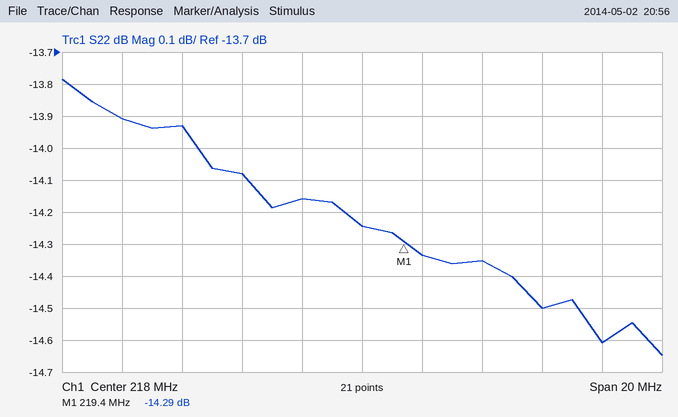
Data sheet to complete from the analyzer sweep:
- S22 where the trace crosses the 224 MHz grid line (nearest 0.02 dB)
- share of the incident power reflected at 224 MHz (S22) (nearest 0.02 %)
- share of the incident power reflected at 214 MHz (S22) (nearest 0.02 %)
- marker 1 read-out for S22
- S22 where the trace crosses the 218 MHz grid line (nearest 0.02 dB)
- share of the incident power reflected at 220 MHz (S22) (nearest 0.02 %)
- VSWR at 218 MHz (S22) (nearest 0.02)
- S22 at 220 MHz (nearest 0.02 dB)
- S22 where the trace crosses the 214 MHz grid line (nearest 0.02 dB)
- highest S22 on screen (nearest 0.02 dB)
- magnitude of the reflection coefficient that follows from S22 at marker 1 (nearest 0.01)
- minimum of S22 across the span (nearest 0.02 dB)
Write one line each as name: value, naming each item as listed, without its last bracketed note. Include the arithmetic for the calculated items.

S22 where the trace crosses the 224 MHz grid line: -14.50 dB
share of the incident power reflected at 224 MHz (S22): 10^(-14.5/10) ≈ 3.55 %, so 3.54 % to the nearest 0.02 %
share of the incident power reflected at 214 MHz (S22): 10^(-14.08/10) ≈ 3.91 %, so 3.90 % to the nearest 0.02 %
marker 1 read-out for S22: -14.29 dB
S22 where the trace crosses the 218 MHz grid line: -14.24 dB
share of the incident power reflected at 220 MHz (S22): 10^(-14.34/10) ≈ 3.68 %
VSWR at 218 MHz (S22): |Γ| = 10^(-14.24/20) = 0.1941; VSWR = (1 + 0.1941)/(1 − 0.1941) ≈ 1.48
S22 at 220 MHz: -14.34 dB
S22 where the trace crosses the 214 MHz grid line: -14.08 dB
highest S22 on screen: -13.78 dB
magnitude of the reflection coefficient that follows from S22 at marker 1: 10^(-14.29/20) ≈ 0.19
minimum of S22 across the span: -14.64 dB
